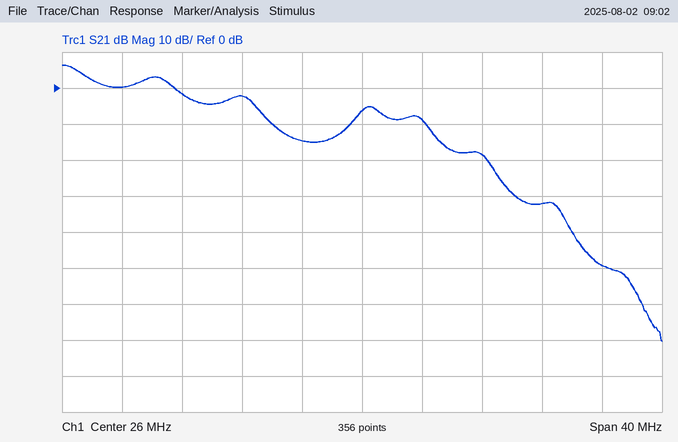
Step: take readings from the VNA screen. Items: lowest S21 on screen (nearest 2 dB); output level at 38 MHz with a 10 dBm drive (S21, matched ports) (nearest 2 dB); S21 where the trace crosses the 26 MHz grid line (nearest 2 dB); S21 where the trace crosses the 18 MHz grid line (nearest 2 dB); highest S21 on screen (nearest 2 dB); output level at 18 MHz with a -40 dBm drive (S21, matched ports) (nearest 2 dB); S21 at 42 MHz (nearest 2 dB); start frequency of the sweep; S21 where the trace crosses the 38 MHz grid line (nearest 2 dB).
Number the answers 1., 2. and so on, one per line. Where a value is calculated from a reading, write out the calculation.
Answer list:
1. -70 dB
2. 10 dBm + (-32 dB) = -22 dBm
3. -6 dB
4. -2 dB
5. 6 dB
6. -40 dBm + (-2 dB) = -42 dBm
7. -50 dB
8. 6 MHz
9. -32 dB
